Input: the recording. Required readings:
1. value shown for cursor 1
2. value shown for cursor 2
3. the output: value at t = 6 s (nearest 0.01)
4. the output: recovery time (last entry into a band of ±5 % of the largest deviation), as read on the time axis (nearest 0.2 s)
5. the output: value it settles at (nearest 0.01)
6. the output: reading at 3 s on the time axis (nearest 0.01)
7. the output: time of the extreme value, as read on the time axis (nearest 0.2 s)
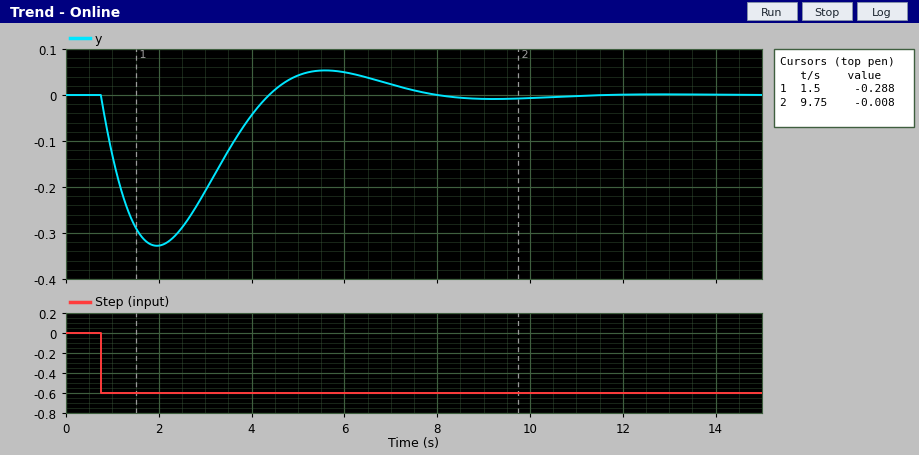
-0.288
-0.008
0.05
7.2 s
0.00
-0.21
2.0 s
